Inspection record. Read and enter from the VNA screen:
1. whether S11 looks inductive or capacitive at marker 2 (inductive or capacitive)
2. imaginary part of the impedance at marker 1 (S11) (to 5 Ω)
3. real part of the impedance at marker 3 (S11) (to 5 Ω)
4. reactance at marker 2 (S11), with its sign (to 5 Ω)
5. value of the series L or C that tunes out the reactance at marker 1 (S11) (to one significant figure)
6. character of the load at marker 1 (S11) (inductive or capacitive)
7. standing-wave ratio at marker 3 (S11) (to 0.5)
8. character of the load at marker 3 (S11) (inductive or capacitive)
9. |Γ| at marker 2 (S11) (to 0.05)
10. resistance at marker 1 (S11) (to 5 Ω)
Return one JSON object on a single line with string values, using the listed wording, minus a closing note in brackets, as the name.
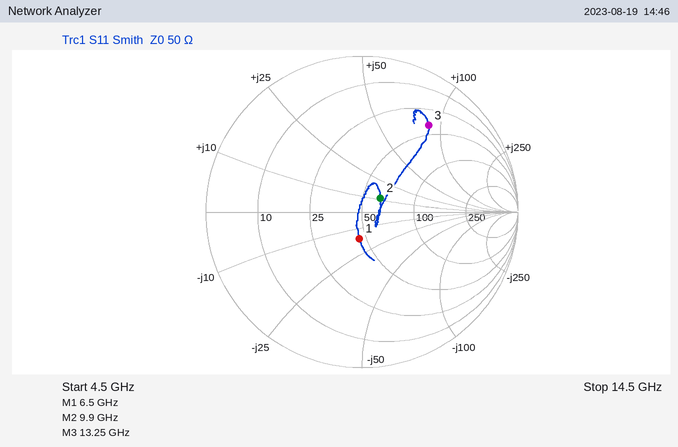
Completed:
{"whether S11 looks inductive or capacitive at marker 2": "inductive", "imaginary part of the impedance at marker 1 (S11)": "-15 Ω", "real part of the impedance at marker 3 (S11)": "40 Ω", "reactance at marker 2 (S11), with its sign": "+10 Ω", "value of the series L or C that tunes out the reactance at marker 1 (S11)": "400 pH", "character of the load at marker 1 (S11)": "capacitive", "standing-wave ratio at marker 3 (S11)": "5.5", "character of the load at marker 3 (S11)": "inductive", "|Γ| at marker 2 (S11)": "0.15", "resistance at marker 1 (S11)": "45 Ω"}
